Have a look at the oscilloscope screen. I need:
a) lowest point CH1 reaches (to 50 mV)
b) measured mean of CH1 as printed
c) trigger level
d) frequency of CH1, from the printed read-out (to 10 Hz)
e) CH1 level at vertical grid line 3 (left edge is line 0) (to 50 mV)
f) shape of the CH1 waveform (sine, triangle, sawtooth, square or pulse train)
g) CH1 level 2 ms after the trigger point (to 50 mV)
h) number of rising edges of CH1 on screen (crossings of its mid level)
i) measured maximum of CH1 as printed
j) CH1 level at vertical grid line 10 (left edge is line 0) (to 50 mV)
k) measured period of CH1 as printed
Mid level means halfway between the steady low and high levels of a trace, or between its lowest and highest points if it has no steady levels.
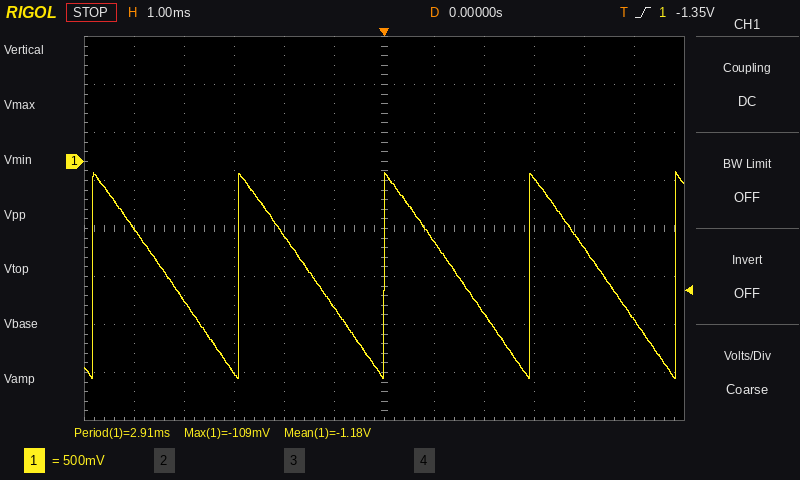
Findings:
-2.25 V
-1.18 V
-1.35 V
340 Hz
-2.20 V
sawtooth
-1.60 V
5
-109 mV
-900 mV
2.91 ms
